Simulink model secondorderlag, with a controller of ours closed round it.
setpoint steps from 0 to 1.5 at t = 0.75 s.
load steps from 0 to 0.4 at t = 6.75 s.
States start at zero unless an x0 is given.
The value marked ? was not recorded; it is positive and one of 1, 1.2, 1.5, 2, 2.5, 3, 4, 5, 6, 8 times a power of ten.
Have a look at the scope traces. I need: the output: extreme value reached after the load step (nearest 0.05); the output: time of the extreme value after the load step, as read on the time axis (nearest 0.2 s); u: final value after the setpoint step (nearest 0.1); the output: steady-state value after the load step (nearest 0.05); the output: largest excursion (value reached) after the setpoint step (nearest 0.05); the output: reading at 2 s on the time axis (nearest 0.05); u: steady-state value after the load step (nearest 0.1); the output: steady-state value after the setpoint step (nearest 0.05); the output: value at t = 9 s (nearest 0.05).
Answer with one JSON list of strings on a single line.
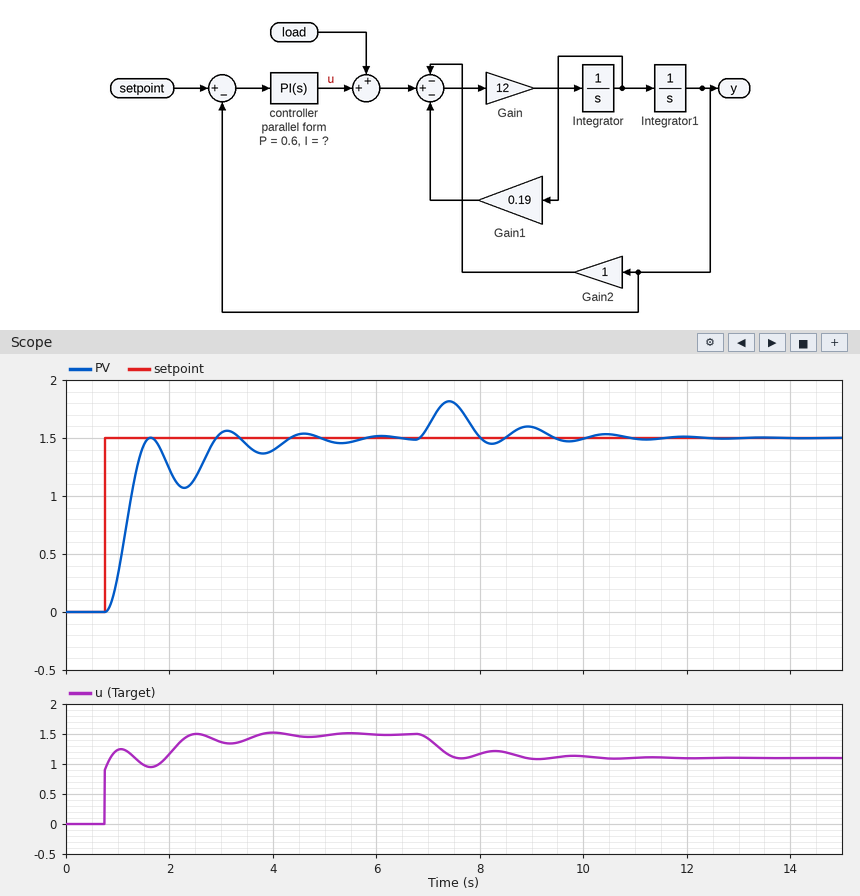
["1.80", "7.4 s", "1.5", "1.50", "1.55", "1.25", "1.1", "1.50", "1.60"]
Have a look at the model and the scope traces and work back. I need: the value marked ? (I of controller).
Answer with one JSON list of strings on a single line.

["1.5"]
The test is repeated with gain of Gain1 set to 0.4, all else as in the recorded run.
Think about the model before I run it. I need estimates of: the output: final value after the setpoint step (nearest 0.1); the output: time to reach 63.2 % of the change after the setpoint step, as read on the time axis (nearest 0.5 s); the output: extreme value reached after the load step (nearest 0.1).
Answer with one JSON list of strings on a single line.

["1.5", "1.5 s", "1.7"]
